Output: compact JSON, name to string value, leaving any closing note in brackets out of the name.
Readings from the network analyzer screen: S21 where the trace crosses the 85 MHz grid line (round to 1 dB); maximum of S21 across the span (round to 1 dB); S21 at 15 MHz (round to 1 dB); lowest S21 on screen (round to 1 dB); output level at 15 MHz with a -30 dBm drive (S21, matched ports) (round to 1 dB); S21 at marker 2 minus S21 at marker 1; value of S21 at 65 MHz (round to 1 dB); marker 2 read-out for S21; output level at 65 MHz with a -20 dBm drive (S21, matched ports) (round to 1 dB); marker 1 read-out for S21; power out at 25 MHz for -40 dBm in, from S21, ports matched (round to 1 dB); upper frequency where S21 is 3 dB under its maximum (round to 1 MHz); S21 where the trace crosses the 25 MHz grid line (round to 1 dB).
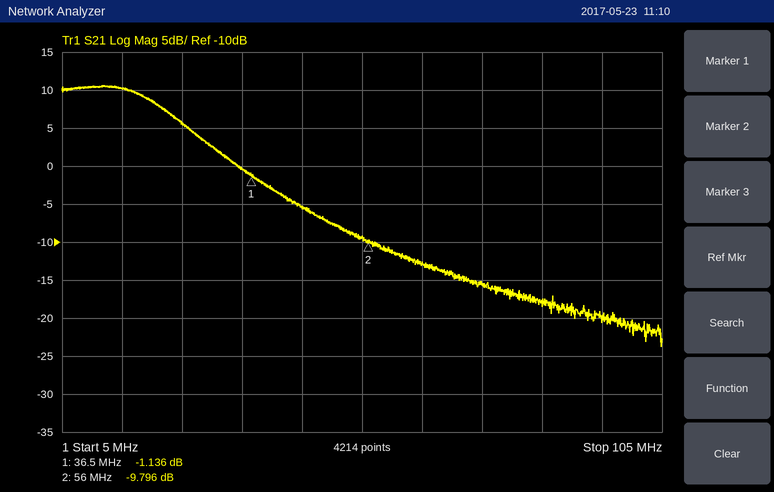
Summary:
{"S21 where the trace crosses the 85 MHz grid line": "-18 dB", "maximum of S21 across the span": "11 dB", "S21 at 15 MHz": "10 dB", "lowest S21 on screen": "-24 dB", "output level at 15 MHz with a -30 dBm drive (S21, matched ports)": "-20 dBm", "S21 at marker 2 minus S21 at marker 1": "-8.660 dB", "value of S21 at 65 MHz": "-13 dB", "marker 2 read-out for S21": "-9.796 dB", "output level at 65 MHz with a -20 dBm drive (S21, matched ports)": "-33 dBm", "marker 1 read-out for S21": "-1.136 dB", "power out at 25 MHz for -40 dBm in, from S21, ports matched": "-34 dBm", "upper frequency where S21 is 3 dB under its maximum": "22 MHz", "S21 where the trace crosses the 25 MHz grid line": "6 dB"}
